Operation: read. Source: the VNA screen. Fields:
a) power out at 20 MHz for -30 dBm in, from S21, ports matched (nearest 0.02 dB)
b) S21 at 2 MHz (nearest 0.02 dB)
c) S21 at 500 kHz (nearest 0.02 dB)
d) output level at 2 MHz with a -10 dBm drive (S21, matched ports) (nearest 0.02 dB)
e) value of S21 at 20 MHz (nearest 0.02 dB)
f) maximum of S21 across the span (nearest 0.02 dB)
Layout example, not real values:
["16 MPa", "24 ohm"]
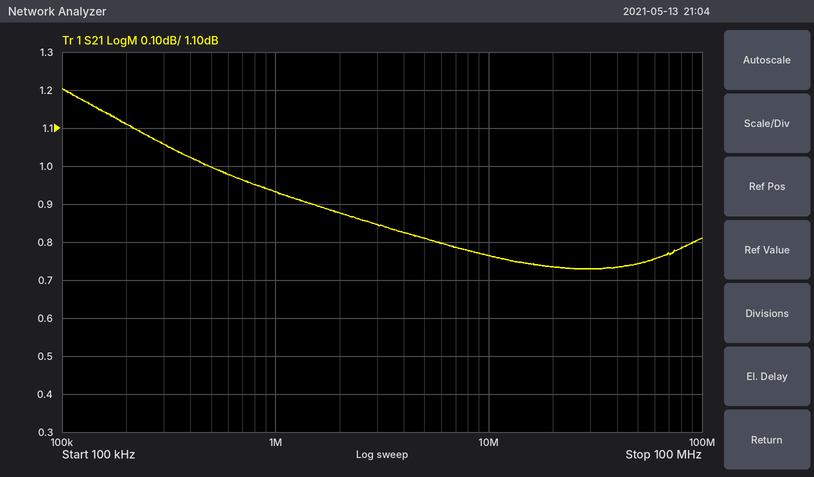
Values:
["-29.26 dBm", "0.88 dB", "1.00 dB", "-9.12 dBm", "0.74 dB", "1.20 dB"]
